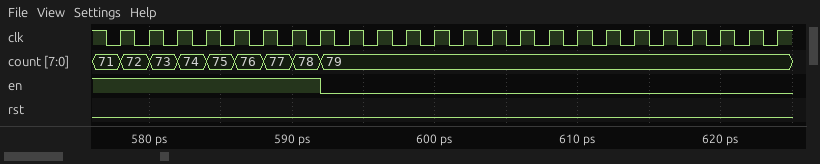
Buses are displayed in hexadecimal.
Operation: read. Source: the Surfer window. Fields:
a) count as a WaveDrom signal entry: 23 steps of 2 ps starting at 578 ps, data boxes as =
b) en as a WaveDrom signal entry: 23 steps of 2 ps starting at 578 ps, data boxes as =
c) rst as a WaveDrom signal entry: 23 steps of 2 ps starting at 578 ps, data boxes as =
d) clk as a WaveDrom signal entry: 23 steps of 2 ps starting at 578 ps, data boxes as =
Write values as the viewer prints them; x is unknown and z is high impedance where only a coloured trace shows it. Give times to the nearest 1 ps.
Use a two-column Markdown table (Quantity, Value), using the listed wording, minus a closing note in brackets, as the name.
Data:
| Quantity | Value |
|---|---|
| count as a WaveDrom signal entry: 23 steps of 2 ps starting at 578 ps, data boxes as = | {name: 'count', wave: '========...............', data: '72 73 74 75 76 77 78 79'} |
| en as a WaveDrom signal entry: 23 steps of 2 ps starting at 578 ps, data boxes as = | {name: 'en', wave: '1......0...............'} |
| rst as a WaveDrom signal entry: 23 steps of 2 ps starting at 578 ps, data boxes as = | {name: 'rst', wave: '0......................'} |
| clk as a WaveDrom signal entry: 23 steps of 2 ps starting at 578 ps, data boxes as = | {name: 'clk', wave: 'p......................'} |
